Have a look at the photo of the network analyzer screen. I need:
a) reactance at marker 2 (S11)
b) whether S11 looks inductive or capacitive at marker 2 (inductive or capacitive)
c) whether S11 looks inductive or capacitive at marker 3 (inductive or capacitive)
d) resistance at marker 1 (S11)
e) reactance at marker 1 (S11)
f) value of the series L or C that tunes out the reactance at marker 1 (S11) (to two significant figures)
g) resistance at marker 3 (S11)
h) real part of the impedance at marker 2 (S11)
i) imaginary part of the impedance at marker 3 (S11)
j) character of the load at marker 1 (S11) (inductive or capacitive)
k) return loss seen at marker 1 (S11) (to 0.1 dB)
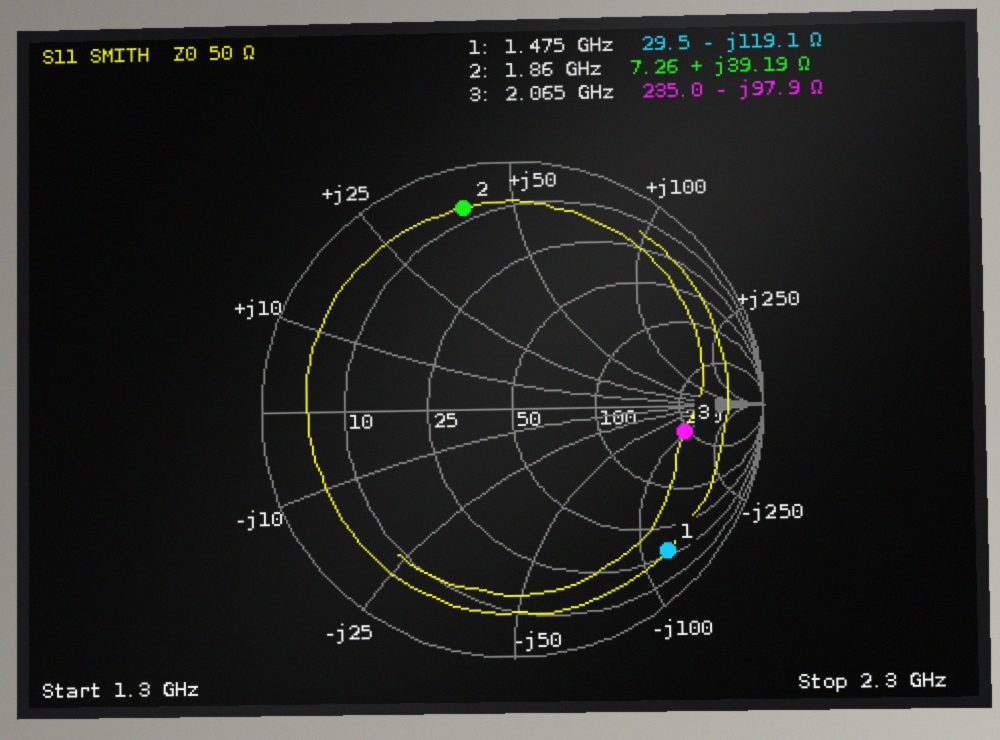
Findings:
+39.19 Ω
inductive
capacitive
29.5 Ω
-119.1 Ω
13 nH
235.0 Ω
7.26 Ω
-97.9 Ω
capacitive
1.5 dB
